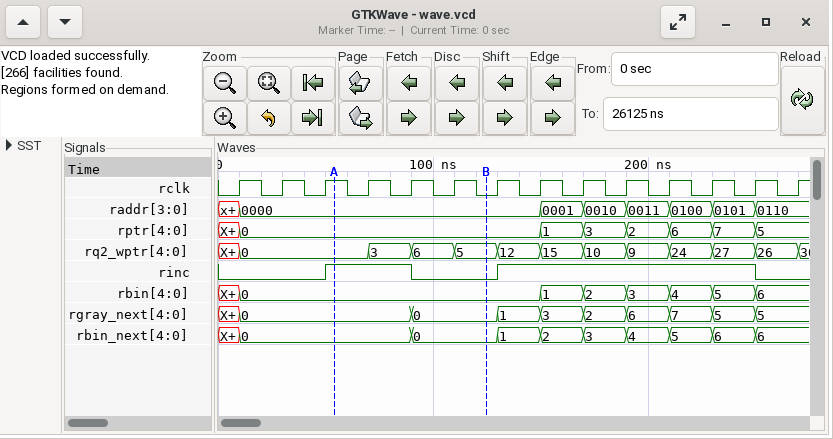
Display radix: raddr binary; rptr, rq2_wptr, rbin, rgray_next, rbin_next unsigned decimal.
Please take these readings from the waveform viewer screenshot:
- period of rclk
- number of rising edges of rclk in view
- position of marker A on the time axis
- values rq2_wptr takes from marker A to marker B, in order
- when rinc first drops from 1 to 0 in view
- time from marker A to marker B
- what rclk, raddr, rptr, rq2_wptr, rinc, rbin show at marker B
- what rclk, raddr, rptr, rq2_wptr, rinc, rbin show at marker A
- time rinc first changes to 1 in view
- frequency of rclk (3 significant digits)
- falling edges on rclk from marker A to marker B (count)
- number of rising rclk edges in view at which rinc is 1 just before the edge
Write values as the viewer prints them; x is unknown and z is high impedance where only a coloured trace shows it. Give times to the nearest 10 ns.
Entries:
20 ns
14
50 ns
0, 3, 6, 5
90 ns
70 ns
rclk=0, raddr=0000, rptr=0, rq2_wptr=5, rinc=0, rbin=0
rclk=1, raddr=0000, rptr=0, rq2_wptr=0, rinc=1, rbin=0
50 ns
50.0 MHz
4
8
